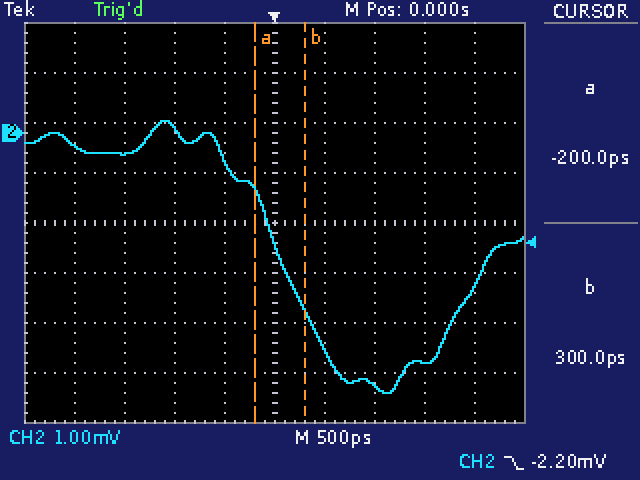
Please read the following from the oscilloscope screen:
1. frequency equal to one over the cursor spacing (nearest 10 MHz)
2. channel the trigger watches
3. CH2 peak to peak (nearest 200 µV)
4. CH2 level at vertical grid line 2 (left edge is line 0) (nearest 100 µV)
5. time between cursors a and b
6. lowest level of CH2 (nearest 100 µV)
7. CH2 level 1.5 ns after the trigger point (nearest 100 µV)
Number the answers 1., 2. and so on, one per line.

1. 2.00 GHz
2. CH2
3. 5.4 mV
4. -400 µV
5. 500 ps
6. -5.2 mV
7. -4.6 mV
